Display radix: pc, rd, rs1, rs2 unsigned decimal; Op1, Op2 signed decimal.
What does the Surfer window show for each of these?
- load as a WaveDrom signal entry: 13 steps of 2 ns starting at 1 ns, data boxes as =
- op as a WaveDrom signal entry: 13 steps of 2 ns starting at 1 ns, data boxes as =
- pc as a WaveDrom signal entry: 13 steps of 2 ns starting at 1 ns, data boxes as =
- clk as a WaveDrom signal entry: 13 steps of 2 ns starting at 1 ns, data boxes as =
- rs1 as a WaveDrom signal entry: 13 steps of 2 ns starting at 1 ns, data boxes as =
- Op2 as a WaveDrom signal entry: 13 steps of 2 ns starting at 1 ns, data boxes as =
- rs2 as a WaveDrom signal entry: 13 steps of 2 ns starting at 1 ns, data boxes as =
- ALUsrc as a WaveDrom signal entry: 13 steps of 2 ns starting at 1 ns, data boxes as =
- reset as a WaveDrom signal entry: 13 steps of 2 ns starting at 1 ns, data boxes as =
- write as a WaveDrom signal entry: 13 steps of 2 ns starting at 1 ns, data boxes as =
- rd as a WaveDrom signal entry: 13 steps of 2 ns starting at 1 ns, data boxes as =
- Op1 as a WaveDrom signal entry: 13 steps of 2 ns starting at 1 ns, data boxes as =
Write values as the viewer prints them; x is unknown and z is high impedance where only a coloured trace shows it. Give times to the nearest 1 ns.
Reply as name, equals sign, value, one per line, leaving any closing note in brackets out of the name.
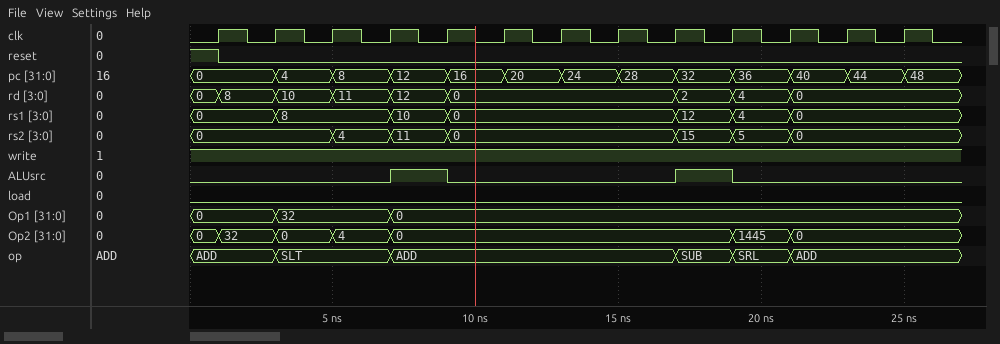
load as a WaveDrom signal entry: 13 steps of 2 ns starting at 1 ns, data boxes as = = {name: 'load', wave: '0............'}
op as a WaveDrom signal entry: 13 steps of 2 ns starting at 1 ns, data boxes as = = {name: 'op', wave: '==.=....===..', data: 'ADD SLT ADD SUB SRL ADD'}
pc as a WaveDrom signal entry: 13 steps of 2 ns starting at 1 ns, data boxes as = = {name: 'pc', wave: '=============', data: '0 4 8 12 16 20 24 28 32 36 40 44 48'}
clk as a WaveDrom signal entry: 13 steps of 2 ns starting at 1 ns, data boxes as = = {name: 'clk', wave: 'p............'}
rs1 as a WaveDrom signal entry: 13 steps of 2 ns starting at 1 ns, data boxes as = = {name: 'rs1', wave: '==.==...===..', data: '0 8 10 0 12 4 0'}
Op2 as a WaveDrom signal entry: 13 steps of 2 ns starting at 1 ns, data boxes as = = {name: 'Op2', wave: '====.....==..', data: '32 0 4 0 1445 0'}
rs2 as a WaveDrom signal entry: 13 steps of 2 ns starting at 1 ns, data boxes as = = {name: 'rs2', wave: '=.===...===..', data: '0 4 11 0 15 5 0'}
ALUsrc as a WaveDrom signal entry: 13 steps of 2 ns starting at 1 ns, data boxes as = = {name: 'ALUsrc', wave: '0..10...10...'}
reset as a WaveDrom signal entry: 13 steps of 2 ns starting at 1 ns, data boxes as = = {name: 'reset', wave: '0............'}
write as a WaveDrom signal entry: 13 steps of 2 ns starting at 1 ns, data boxes as = = {name: 'write', wave: '1............'}
rd as a WaveDrom signal entry: 13 steps of 2 ns starting at 1 ns, data boxes as = = {name: 'rd', wave: '=====...===..', data: '8 10 11 12 0 2 4 0'}
Op1 as a WaveDrom signal entry: 13 steps of 2 ns starting at 1 ns, data boxes as = = {name: 'Op1', wave: '==.=.........', data: '0 32 0'}
